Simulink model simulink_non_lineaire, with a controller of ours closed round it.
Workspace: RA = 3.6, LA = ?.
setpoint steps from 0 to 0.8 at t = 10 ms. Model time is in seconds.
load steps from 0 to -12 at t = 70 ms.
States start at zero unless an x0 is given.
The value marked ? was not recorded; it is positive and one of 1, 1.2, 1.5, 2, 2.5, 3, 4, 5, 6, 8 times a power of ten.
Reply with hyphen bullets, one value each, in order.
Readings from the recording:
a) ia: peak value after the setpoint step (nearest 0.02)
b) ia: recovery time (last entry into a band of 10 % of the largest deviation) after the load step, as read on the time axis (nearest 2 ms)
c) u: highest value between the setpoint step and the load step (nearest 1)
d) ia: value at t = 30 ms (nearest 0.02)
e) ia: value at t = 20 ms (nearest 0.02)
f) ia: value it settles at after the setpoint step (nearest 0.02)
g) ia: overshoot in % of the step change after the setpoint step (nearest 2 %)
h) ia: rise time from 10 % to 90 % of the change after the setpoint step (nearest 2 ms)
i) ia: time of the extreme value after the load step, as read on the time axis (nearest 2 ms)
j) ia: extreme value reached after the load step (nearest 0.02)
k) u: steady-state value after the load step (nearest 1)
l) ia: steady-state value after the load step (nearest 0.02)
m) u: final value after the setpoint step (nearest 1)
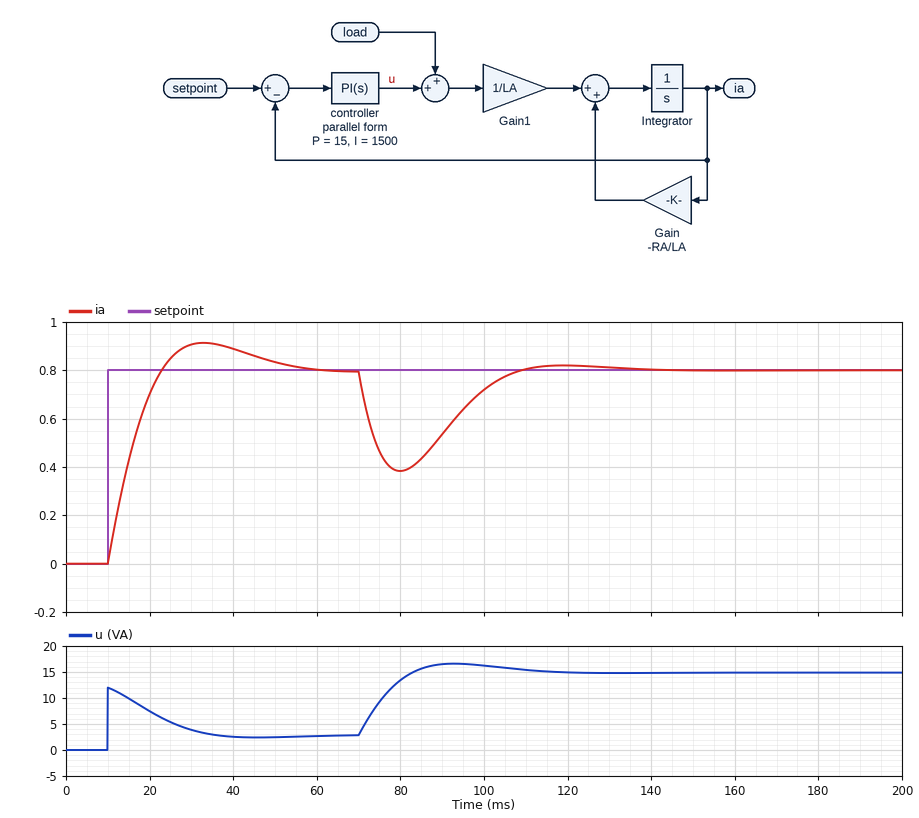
- 0.92
- 104 ms
- 12
- 0.90
- 0.70
- 0.80
- 14 %
- 10 ms
- 80 ms
- 0.38
- 15
- 0.80
- 3
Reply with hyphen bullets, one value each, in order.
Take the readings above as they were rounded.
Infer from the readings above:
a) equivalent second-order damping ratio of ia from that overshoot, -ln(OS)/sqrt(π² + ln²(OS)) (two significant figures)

- 0.53
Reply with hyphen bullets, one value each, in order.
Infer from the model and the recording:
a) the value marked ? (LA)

- 0.12
